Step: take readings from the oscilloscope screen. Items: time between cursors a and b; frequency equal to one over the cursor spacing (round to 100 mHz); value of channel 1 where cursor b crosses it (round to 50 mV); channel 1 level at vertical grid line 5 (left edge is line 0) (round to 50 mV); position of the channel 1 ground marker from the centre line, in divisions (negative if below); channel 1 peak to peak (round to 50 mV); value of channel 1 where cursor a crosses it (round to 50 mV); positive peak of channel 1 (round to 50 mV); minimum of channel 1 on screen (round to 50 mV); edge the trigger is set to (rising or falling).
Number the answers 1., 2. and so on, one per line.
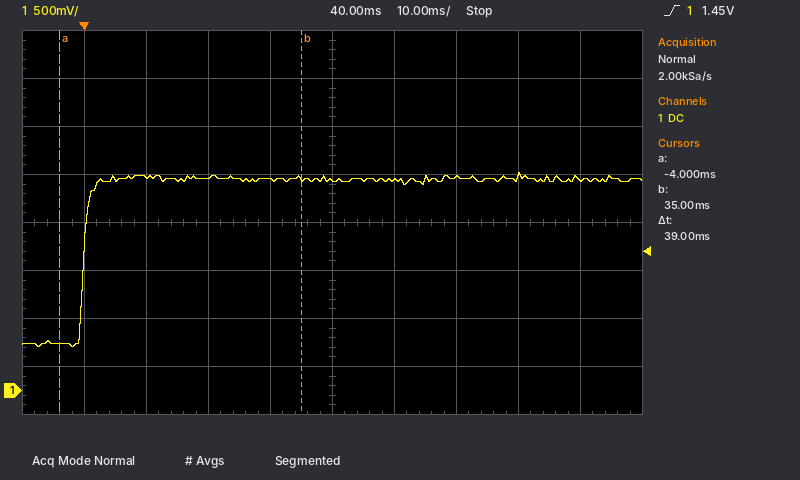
1. 39 ms
2. 25.6 Hz
3. 2.20 V
4. 2.20 V
5. -3.5 div
6. 1.80 V
7. 500 mV
8. 2.25 V
9. 450 mV
10. rising
